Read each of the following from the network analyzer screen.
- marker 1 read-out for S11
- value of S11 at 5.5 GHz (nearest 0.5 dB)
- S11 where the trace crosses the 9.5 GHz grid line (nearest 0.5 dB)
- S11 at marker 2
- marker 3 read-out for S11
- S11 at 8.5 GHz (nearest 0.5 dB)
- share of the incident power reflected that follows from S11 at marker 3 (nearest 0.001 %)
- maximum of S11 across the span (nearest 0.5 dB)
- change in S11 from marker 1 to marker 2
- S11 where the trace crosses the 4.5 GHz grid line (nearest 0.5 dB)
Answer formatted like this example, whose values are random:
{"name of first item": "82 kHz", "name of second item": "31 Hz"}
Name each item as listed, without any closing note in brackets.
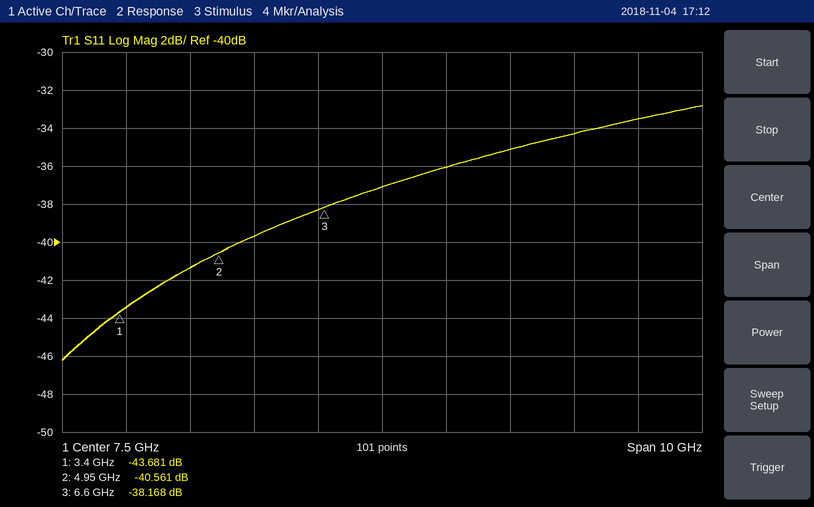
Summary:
{"marker 1 read-out for S11": "-43.681 dB", "value of S11 at 5.5 GHz": "-39.5 dB", "S11 where the trace crosses the 9.5 GHz grid line": "-35.0 dB", "S11 at marker 2": "-40.561 dB", "marker 3 read-out for S11": "-38.168 dB", "S11 at 8.5 GHz": "-36.0 dB", "share of the incident power reflected that follows from S11 at marker 3": "0.015 %", "maximum of S11 across the span": "-33.0 dB", "change in S11 from marker 1 to marker 2": "3.120 dB", "S11 where the trace crosses the 4.5 GHz grid line": "-41.5 dB"}
